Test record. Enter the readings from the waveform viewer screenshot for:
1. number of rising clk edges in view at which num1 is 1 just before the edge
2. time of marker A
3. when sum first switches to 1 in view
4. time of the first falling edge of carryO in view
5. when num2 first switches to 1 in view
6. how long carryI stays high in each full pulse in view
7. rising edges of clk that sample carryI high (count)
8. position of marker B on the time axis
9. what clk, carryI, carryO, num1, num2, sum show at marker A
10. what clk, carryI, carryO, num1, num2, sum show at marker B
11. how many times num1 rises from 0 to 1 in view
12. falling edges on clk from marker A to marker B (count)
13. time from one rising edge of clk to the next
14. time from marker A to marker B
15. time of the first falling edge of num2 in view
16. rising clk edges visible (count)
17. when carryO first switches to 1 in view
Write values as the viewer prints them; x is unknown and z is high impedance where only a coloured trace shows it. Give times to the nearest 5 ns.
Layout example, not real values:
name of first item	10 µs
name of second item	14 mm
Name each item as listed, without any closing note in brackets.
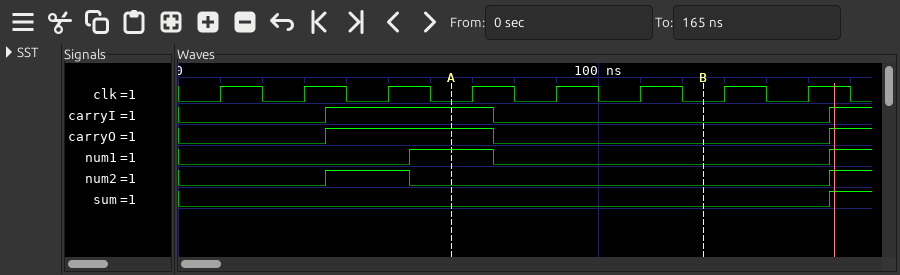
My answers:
number of rising clk edges in view at which num1 is 1 just before the edge	1
time of marker A	65 ns
when sum first switches to 1 in view	155 ns
time of the first falling edge of carryO in view	75 ns
when num2 first switches to 1 in view	35 ns
how long carryI stays high in each full pulse in view	40 ns
rising edges of clk that sample carryI high	2
position of marker B on the time axis	125 ns
what clk, carryI, carryO, num1, num2, sum show at marker A	clk=0, carryI=1, carryO=1, num1=1, num2=0, sum=0
what clk, carryI, carryO, num1, num2, sum show at marker B	clk=0, carryI=0, carryO=0, num1=0, num2=0, sum=0
how many times num1 rises from 0 to 1 in view	2
falling edges on clk from marker A to marker B	3
time from one rising edge of clk to the next	20 ns
time from marker A to marker B	60 ns
time of the first falling edge of num2 in view	55 ns
rising clk edges visible	8
when carryO first switches to 1 in view	35 ns
